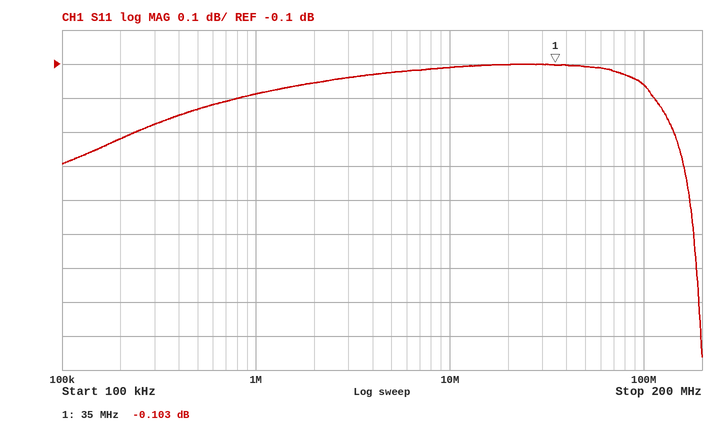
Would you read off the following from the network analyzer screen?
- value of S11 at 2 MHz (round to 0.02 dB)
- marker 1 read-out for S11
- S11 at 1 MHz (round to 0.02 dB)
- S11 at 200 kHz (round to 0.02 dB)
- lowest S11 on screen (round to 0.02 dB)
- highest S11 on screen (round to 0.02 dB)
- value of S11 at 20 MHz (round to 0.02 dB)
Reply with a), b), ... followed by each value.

a) -0.16 dB
b) -0.103 dB
c) -0.18 dB
d) -0.32 dB
e) -0.96 dB
f) -0.10 dB
g) -0.10 dB
